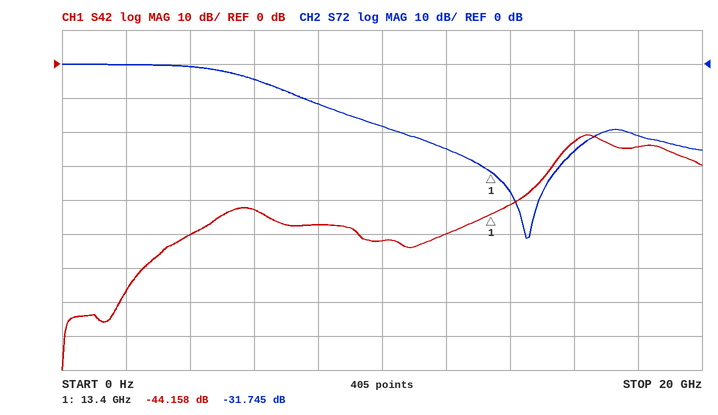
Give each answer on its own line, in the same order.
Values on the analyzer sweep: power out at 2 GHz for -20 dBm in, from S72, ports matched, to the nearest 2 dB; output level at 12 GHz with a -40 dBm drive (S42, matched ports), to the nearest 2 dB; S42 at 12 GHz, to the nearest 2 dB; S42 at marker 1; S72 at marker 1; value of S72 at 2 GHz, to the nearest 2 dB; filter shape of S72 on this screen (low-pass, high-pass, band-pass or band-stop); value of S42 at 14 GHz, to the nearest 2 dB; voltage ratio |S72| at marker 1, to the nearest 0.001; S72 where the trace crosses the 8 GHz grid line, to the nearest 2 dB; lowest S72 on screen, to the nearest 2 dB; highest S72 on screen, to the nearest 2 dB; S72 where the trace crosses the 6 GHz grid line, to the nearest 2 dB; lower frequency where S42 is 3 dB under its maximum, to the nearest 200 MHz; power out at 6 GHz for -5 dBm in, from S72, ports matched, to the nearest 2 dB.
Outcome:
-20 dBm
-90 dBm
-50 dB
-44.158 dB
-31.745 dB
0 dB
low-pass
-42 dB
0.026
-12 dB
-52 dB
0 dB
-4 dB
15.8 GHz
-10 dBm
